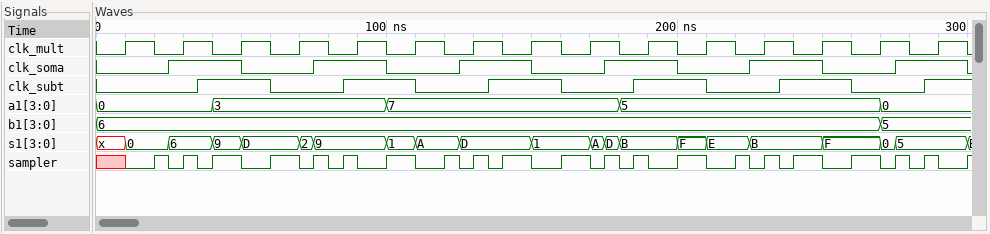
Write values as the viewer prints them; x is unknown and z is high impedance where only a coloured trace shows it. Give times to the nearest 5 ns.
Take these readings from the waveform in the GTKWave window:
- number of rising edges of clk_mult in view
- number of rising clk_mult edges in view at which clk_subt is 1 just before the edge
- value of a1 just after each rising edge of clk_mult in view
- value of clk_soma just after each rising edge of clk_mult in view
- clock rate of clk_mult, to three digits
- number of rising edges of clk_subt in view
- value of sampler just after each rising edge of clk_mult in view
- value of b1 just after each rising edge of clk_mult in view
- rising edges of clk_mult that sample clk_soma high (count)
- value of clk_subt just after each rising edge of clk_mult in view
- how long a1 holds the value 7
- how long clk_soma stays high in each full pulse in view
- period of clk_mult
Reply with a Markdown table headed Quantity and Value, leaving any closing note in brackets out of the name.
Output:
| Quantity | Value |
|---|---|
| number of rising edges of clk_mult in view | 15 |
| number of rising clk_mult edges in view at which clk_subt is 1 just before the edge | 8 |
| value of a1 just after each rising edge of clk_mult in view | 0, 0, 3, 3, 3, 7, 7, 7, 7, 5, 5, 5, 5, 0, 0 |
| value of clk_soma just after each rising edge of clk_mult in view | 0 1 0 0 1 0 1 0 0 1 0 1 0 0 1 |
| clock rate of clk_mult, to three digits | 50.0 MHz |
| number of rising edges of clk_subt in view | 6 |
| value of sampler just after each rising edge of clk_mult in view | 0 1 0 0 0 0 1 0 0 0 0 1 0 0 0 |
| value of b1 just after each rising edge of clk_mult in view | 6, 6, 6, 6, 6, 6, 6, 6, 6, 6, 6, 6, 6, 5, 5 |
| rising edges of clk_mult that sample clk_soma high | 9 |
| value of clk_subt just after each rising edge of clk_mult in view | 0 0 1 0 1 0 0 1 0 1 0 0 1 0 1 |
| how long a1 holds the value 7 | 80 ns |
| how long clk_soma stays high in each full pulse in view | 25 ns, 25 ns, 25 ns, 25 ns, 25 ns, 25 ns |
| period of clk_mult | 20 ns |
